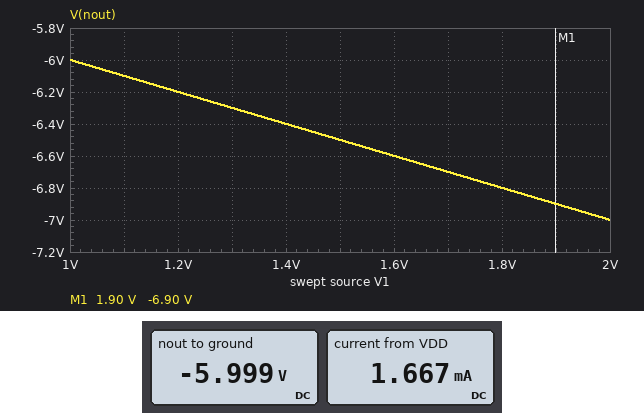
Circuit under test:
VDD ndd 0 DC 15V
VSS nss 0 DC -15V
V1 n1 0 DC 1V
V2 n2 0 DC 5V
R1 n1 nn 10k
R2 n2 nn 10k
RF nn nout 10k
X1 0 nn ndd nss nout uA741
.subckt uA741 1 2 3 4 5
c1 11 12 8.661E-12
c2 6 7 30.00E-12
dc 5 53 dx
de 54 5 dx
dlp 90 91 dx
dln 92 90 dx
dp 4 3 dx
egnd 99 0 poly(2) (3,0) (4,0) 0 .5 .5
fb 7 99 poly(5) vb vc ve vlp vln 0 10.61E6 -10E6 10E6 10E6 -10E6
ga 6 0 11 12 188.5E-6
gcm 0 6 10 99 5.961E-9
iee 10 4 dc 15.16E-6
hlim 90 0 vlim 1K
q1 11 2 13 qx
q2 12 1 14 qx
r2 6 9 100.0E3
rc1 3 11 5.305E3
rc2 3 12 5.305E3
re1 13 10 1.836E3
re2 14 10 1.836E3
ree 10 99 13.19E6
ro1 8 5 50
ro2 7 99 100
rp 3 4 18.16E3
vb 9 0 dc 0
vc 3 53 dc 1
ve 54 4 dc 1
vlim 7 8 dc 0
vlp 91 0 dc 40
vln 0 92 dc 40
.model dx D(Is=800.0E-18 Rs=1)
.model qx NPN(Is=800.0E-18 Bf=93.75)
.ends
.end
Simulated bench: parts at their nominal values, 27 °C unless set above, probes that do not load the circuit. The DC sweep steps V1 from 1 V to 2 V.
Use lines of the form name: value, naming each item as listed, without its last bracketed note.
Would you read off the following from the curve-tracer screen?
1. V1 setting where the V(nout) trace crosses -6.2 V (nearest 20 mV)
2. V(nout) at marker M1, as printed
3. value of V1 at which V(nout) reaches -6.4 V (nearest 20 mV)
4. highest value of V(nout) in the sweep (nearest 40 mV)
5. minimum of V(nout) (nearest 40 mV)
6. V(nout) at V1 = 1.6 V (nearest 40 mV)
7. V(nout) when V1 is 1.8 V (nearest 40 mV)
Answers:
V1 setting where the V(nout) trace crosses -6.2 V: 1.20 V
V(nout) at marker M1, as printed: -6.90 V
value of V1 at which V(nout) reaches -6.4 V: 1.40 V
highest value of V(nout) in the sweep: -6.00 V
minimum of V(nout): -7.00 V
V(nout) at V1 = 1.6 V: -6.60 V
V(nout) when V1 is 1.8 V: -6.80 V
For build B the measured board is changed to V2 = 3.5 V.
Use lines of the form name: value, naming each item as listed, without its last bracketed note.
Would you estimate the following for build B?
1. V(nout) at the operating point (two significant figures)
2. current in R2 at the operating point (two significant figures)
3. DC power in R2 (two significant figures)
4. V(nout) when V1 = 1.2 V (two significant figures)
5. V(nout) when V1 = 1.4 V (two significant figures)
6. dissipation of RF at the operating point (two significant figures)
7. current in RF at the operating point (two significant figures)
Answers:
V(nout) at the operating point: -4.5 V
current in R2 at the operating point: 350 µA
DC power in R2: 1.2 mW
V(nout) when V1 = 1.2 V: -4.7 V
V(nout) when V1 = 1.4 V: -4.9 V
dissipation of RF at the operating point: 2.0 mW
current in RF at the operating point: 450 µA
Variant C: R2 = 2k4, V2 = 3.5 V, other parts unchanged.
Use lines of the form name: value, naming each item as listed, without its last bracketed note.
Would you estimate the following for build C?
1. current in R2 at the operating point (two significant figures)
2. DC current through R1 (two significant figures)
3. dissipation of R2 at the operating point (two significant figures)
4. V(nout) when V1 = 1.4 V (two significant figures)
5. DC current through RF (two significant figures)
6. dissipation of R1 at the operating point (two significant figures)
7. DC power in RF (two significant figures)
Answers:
current in R2 at the operating point: 1.4 mA
DC current through R1: 84 µA
dissipation of R2 at the operating point: 4.7 mW
V(nout) when V1 = 1.4 V: -15 V
DC current through RF: 1.5 mA
dissipation of R1 at the operating point: 71 µW
DC power in RF: 22 mW
